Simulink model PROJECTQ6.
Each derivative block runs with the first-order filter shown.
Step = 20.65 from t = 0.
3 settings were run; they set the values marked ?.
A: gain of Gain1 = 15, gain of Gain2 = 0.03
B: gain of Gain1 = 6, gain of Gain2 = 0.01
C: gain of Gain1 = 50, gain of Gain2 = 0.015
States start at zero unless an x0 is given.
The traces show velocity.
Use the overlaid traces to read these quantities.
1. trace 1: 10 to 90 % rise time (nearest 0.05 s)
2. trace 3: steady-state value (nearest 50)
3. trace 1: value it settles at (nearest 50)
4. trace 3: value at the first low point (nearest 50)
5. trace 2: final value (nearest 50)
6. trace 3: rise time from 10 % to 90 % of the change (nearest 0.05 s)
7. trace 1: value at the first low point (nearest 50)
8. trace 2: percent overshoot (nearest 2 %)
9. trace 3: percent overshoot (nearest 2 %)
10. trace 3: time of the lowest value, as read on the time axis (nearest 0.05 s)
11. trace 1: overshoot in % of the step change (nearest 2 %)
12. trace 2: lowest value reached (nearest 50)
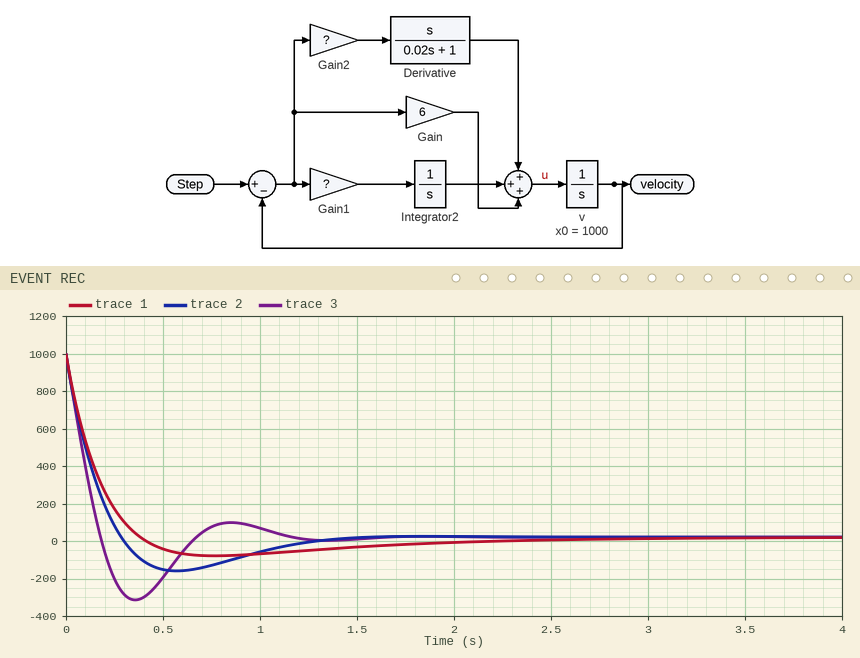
0.25 s
0
0
-300
0
0.15 s
-100
18 %
34 %
0.35 s
10 %
-150
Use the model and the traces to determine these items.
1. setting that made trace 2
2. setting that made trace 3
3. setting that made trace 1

A
C
B
